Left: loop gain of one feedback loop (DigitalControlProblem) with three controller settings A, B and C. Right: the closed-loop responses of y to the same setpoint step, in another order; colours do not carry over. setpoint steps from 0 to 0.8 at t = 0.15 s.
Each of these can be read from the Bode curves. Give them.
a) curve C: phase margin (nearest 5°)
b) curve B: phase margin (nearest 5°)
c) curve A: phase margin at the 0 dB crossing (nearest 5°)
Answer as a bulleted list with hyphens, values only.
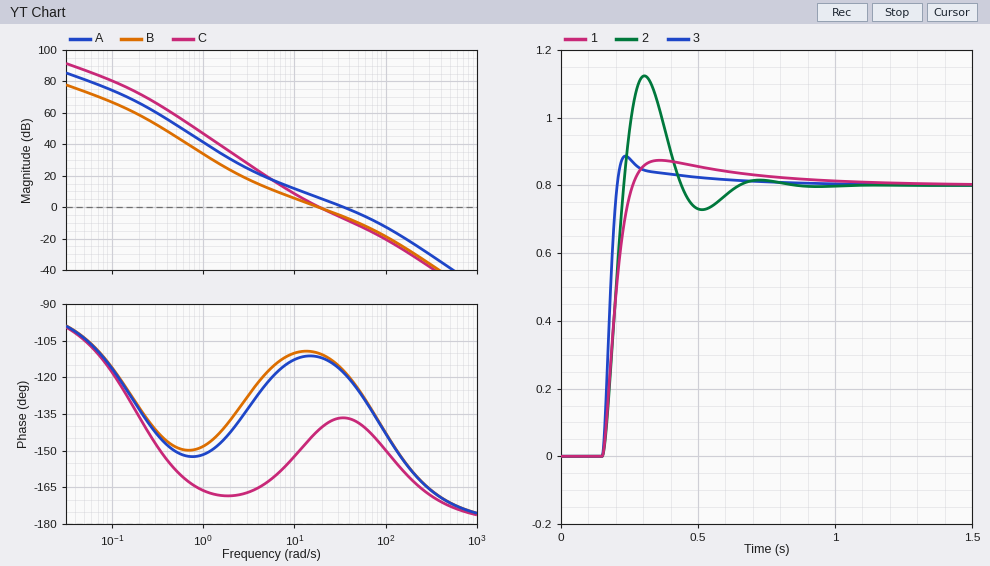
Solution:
- 40°
- 70°
- 60°
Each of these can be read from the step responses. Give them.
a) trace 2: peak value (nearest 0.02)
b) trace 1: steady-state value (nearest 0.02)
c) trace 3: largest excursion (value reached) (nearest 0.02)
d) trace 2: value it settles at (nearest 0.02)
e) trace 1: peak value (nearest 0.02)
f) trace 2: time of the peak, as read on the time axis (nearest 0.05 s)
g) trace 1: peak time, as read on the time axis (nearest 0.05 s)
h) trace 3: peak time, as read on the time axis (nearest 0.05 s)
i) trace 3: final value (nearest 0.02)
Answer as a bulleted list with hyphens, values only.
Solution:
- 1.12
- 0.80
- 0.88
- 0.80
- 0.88
- 0.30 s
- 0.35 s
- 0.25 s
- 0.80
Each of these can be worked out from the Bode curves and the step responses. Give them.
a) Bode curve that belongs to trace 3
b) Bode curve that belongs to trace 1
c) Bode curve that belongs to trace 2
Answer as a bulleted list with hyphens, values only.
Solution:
- A
- B
- C
